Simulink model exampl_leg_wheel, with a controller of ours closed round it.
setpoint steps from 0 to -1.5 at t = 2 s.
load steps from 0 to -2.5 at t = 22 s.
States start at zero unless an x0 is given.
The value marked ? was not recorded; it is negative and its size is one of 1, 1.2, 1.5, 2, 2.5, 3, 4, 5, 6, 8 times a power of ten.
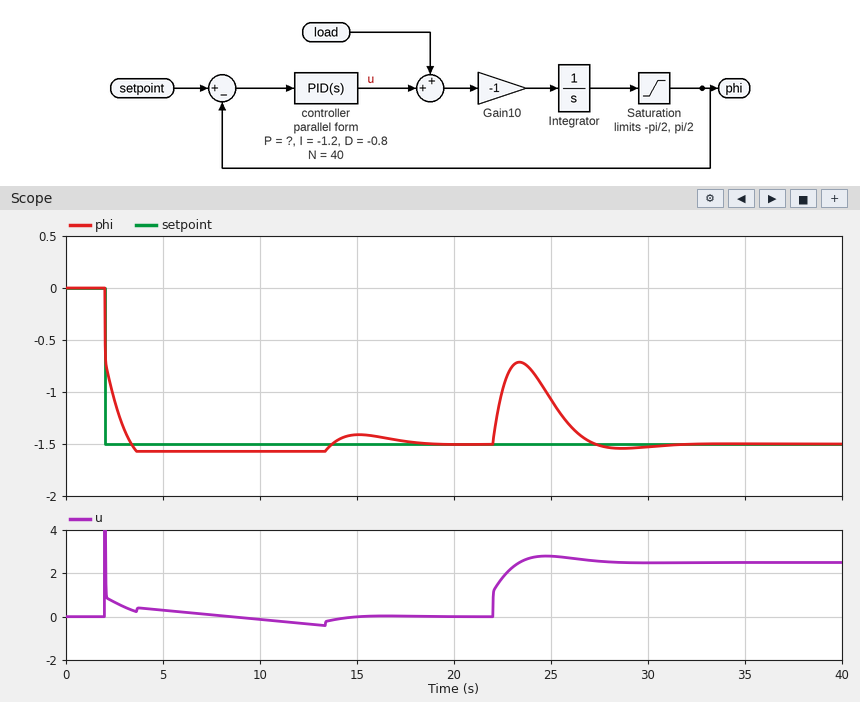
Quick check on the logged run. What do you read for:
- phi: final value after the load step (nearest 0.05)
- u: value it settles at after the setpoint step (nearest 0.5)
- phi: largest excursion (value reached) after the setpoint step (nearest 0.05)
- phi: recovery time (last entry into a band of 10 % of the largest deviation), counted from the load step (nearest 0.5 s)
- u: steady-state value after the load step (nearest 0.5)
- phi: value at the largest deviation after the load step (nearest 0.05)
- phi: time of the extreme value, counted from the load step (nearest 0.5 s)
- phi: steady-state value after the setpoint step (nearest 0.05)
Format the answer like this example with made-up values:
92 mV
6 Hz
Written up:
-1.50
0.0
-1.55
4.5 s
2.5
-0.70
1.5 s
-1.50
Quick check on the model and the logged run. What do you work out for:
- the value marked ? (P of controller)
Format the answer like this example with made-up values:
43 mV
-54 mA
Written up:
-2
